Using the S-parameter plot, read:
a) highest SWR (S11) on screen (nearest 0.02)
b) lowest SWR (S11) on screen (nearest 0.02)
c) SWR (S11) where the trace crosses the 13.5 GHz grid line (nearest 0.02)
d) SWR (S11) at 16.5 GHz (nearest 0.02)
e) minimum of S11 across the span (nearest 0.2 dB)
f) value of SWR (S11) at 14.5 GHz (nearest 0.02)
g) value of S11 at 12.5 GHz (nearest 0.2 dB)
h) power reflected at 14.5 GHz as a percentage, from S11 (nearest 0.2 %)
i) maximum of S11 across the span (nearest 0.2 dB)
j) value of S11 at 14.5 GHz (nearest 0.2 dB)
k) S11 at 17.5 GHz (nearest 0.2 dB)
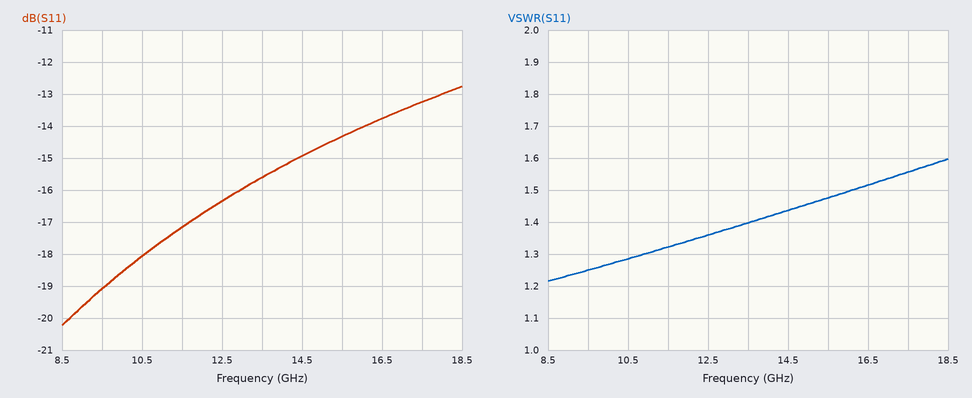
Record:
1.60
1.22
1.40
1.52
-20.2 dB
1.44
-16.4 dB
3.2 %
-12.8 dB
-15.0 dB
-13.2 dB
